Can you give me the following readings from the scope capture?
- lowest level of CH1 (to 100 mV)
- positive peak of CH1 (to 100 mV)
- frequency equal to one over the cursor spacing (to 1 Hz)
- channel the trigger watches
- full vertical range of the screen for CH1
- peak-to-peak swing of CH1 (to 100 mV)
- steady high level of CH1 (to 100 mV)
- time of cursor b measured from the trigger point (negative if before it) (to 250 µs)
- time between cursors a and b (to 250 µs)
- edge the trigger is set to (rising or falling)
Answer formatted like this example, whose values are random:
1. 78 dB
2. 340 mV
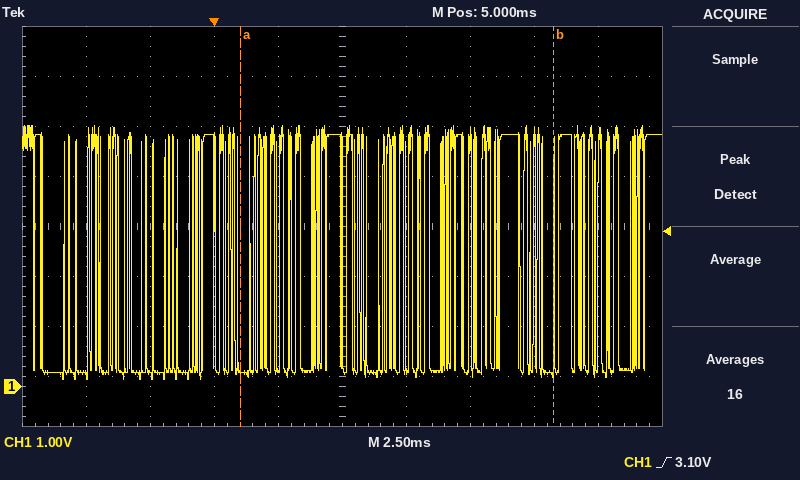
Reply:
1. 100 mV
2. 5.2 V
3. 82 Hz
4. CH1
5. 8 V
6. 5.1 V
7. 5.0 V
8. +13.25 ms
9. 12.25 ms
10. rising
